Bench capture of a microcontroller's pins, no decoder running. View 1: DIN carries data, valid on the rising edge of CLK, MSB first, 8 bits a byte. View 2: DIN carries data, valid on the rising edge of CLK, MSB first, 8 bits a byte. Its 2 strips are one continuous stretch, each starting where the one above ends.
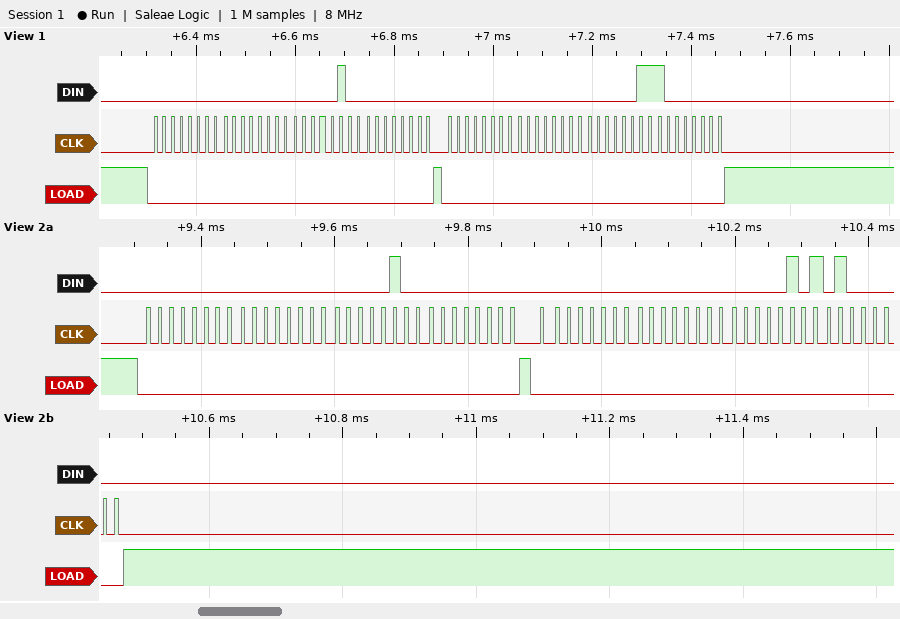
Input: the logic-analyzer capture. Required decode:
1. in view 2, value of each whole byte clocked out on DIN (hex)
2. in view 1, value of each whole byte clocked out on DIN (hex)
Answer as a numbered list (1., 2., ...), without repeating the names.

1. 00 00 04 00 00 00 05 40
2. 0x00 0x00 0x04 0x00 0x00 0x00 0x03 0x80
